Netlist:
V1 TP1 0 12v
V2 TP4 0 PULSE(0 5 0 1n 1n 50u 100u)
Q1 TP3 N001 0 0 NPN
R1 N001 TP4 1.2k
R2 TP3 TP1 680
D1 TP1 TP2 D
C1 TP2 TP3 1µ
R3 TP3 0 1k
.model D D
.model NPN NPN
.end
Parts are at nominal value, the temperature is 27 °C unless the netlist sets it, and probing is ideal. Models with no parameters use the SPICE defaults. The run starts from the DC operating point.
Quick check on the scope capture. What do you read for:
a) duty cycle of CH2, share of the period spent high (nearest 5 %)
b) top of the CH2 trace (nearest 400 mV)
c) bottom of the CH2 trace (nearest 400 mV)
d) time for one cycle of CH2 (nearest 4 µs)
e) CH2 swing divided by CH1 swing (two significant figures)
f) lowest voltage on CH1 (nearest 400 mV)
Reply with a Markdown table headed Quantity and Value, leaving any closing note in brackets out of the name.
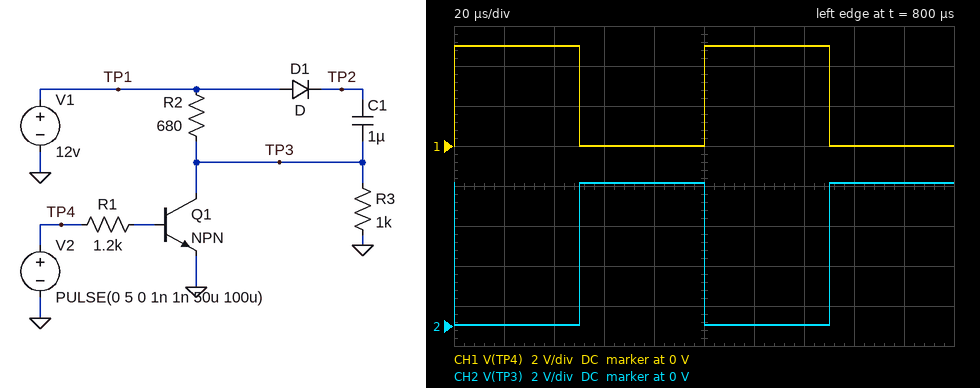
| Quantity | Value |
|---|---|
| duty cycle of CH2, share of the period spent high | 50 % |
| top of the CH2 trace | 7.2 V |
| bottom of the CH2 trace | 0 V |
| time for one cycle of CH2 | 100 µs |
| CH2 swing divided by CH1 swing | 1.4 |
| lowest voltage on CH1 | 0 V |
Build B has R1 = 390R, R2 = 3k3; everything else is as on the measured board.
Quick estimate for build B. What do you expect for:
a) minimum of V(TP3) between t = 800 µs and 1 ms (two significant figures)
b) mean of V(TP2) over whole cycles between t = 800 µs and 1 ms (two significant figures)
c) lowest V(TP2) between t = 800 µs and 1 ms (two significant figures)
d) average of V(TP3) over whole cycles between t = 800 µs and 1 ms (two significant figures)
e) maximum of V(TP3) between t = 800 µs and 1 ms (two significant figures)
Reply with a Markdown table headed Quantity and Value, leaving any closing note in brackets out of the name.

| Quantity | Value |
|---|---|
| minimum of V(TP3) between t = 800 µs and 1 ms | 22 mV |
| mean of V(TP2) over whole cycles between t = 800 µs and 1 ms | 13 V |
| lowest V(TP2) between t = 800 µs and 1 ms | 11 V |
| average of V(TP3) over whole cycles between t = 800 µs and 1 ms | 1.4 V |
| maximum of V(TP3) between t = 800 µs and 1 ms | 2.8 V |
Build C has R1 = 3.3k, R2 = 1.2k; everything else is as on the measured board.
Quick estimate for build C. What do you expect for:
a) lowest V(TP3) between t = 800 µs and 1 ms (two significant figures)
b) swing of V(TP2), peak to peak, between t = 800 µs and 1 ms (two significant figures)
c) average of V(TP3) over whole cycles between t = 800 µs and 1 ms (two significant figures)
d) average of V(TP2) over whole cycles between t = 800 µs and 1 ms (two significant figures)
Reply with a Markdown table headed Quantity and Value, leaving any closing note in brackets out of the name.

| Quantity | Value |
|---|---|
| lowest V(TP3) between t = 800 µs and 1 ms | 61 mV |
| swing of V(TP2), peak to peak, between t = 800 µs and 1 ms | 5.4 V |
| average of V(TP3) over whole cycles between t = 800 µs and 1 ms | 2.8 V |
| average of V(TP2) over whole cycles between t = 800 µs and 1 ms | 14 V |
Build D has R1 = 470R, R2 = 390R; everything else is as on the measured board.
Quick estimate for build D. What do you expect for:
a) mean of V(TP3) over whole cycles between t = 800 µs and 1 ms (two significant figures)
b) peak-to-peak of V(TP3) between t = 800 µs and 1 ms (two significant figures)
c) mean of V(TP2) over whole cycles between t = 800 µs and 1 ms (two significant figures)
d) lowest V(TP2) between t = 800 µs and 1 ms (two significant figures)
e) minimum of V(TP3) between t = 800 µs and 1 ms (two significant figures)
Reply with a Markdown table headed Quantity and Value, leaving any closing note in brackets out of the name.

| Quantity | Value |
|---|---|
| mean of V(TP3) over whole cycles between t = 800 µs and 1 ms | 4.3 V |
| peak-to-peak of V(TP3) between t = 800 µs and 1 ms | 8.6 V |
| mean of V(TP2) over whole cycles between t = 800 µs and 1 ms | 16 V |
| lowest V(TP2) between t = 800 µs and 1 ms | 11 V |
| minimum of V(TP3) between t = 800 µs and 1 ms | 45 mV |
